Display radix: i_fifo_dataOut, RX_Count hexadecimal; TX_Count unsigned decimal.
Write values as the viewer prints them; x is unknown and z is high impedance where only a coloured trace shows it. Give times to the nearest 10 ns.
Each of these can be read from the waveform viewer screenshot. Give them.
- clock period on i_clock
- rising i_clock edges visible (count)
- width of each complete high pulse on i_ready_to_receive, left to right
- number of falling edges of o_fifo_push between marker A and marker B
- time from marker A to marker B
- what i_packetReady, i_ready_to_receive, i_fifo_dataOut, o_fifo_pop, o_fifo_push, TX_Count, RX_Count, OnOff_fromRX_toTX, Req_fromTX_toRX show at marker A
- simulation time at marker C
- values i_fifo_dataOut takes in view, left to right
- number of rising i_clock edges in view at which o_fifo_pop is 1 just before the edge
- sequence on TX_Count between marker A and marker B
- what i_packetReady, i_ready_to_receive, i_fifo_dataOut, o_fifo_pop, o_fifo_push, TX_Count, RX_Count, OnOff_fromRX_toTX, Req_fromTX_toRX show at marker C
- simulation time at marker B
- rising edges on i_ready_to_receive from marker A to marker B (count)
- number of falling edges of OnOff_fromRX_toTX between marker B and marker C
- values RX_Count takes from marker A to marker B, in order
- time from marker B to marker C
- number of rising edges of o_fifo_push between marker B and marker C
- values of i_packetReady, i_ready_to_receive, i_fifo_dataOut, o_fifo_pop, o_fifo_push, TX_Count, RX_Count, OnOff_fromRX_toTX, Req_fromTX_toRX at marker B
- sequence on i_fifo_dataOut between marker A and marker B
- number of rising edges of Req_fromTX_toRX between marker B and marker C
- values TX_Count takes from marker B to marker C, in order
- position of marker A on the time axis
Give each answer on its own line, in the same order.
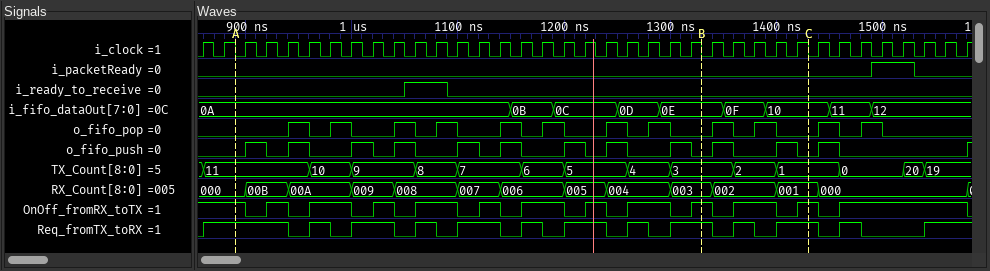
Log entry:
20 ns
37
40 ns
9
440 ns
i_packetReady=0, i_ready_to_receive=0, i_fifo_dataOut=0A, o_fifo_pop=0, o_fifo_push=0, TX_Count=11, RX_Count=000, OnOff_fromRX_toTX=1, Req_fromTX_toRX=1
1430 ns
0A, 0B, 0C, 0D, 0E, 0F, 10, 11, 12
12
11, 10, 9, 8, 7, 6, 5, 4, 3
i_packetReady=0, i_ready_to_receive=0, i_fifo_dataOut=10, o_fifo_pop=0, o_fifo_push=0, TX_Count=1, RX_Count=001, OnOff_fromRX_toTX=1, Req_fromTX_toRX=1
1330 ns
1
2
000, 00B, 00A, 009, 008, 007, 006, 005, 004, 003
100 ns
2
i_packetReady=0, i_ready_to_receive=0, i_fifo_dataOut=0E, o_fifo_pop=0, o_fifo_push=0, TX_Count=3, RX_Count=003, OnOff_fromRX_toTX=1, Req_fromTX_toRX=1
0A, 0B, 0C, 0D, 0E
2
3, 2, 1
890 ns
